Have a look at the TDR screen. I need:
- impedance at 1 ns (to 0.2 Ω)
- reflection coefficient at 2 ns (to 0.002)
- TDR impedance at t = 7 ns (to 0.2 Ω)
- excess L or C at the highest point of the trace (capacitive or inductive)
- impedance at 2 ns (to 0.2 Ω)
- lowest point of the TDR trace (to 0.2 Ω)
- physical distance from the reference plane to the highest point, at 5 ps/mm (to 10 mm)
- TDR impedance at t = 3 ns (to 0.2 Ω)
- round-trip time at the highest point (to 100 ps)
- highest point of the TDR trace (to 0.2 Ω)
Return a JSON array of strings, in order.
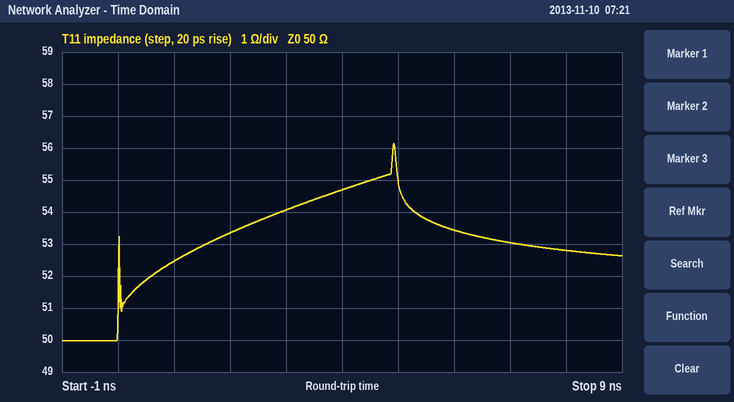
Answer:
["52.4 Ω", "+0.032", "53.0 Ω", "inductive", "53.4 Ω", "50.0 Ω", "490 mm", "54.0 Ω", "4.9 ns", "56.2 Ω"]
